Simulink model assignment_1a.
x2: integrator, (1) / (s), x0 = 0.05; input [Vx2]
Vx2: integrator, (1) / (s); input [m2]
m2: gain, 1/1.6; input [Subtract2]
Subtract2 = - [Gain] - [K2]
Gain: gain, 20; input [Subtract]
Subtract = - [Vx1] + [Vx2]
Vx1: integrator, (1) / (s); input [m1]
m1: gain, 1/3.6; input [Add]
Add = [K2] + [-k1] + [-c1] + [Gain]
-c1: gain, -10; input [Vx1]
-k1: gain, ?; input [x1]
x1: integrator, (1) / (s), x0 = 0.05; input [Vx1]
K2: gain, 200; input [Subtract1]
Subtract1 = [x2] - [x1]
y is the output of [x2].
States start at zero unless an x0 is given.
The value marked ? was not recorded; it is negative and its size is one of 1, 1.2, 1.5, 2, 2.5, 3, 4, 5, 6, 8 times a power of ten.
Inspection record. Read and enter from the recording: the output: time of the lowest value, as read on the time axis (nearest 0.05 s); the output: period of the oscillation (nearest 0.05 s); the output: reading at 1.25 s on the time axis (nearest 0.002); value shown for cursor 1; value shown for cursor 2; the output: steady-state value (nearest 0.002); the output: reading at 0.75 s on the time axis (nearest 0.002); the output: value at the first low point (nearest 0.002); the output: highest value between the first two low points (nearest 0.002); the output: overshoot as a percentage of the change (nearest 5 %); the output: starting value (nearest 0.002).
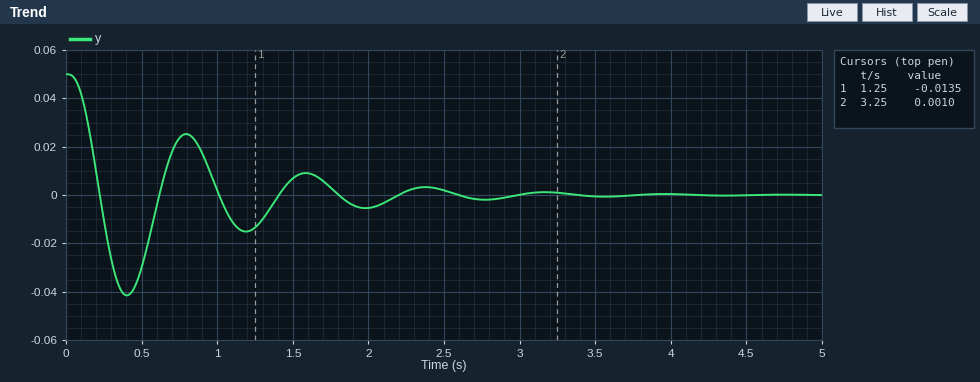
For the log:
0.40 s
0.80 s
-0.014
-0.0135
0.0010
0.000
0.024
-0.042
0.026
85 %
0.050
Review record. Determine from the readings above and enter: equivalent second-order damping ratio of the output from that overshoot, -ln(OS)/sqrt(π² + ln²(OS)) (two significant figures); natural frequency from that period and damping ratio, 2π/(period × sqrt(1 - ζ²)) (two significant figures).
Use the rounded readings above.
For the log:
0.052
7.9 rad/s
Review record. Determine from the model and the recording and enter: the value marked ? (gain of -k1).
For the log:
-400
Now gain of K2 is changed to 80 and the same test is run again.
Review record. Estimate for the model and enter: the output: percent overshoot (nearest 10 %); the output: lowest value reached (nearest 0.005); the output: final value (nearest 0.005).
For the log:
70 %
-0.035
0.000
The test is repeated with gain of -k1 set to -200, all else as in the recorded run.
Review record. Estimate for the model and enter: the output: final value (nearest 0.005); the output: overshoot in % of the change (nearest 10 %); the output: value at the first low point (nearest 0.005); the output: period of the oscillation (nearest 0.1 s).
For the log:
0.000
70 %
-0.035
1.1 s
